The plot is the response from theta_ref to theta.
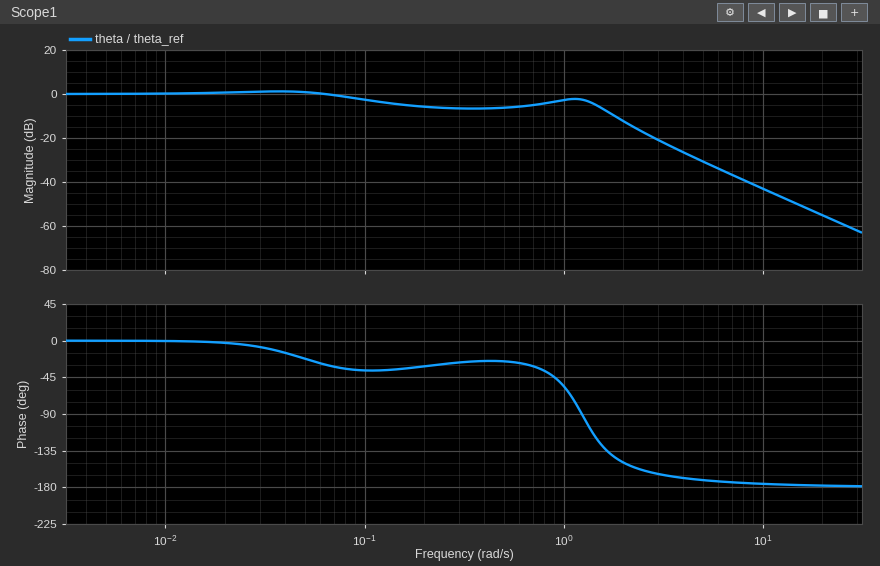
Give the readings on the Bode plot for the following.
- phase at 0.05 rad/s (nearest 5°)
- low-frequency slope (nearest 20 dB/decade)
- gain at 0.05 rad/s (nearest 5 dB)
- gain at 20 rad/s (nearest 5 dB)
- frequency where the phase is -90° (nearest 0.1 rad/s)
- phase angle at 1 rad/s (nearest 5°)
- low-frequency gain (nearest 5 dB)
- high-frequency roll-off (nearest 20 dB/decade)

-20°
0 dB/decade
0 dB
-55 dB
1.2 rad/s
-55°
0 dB
-40 dB/decade
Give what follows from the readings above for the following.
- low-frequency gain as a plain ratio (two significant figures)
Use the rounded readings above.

1.0
